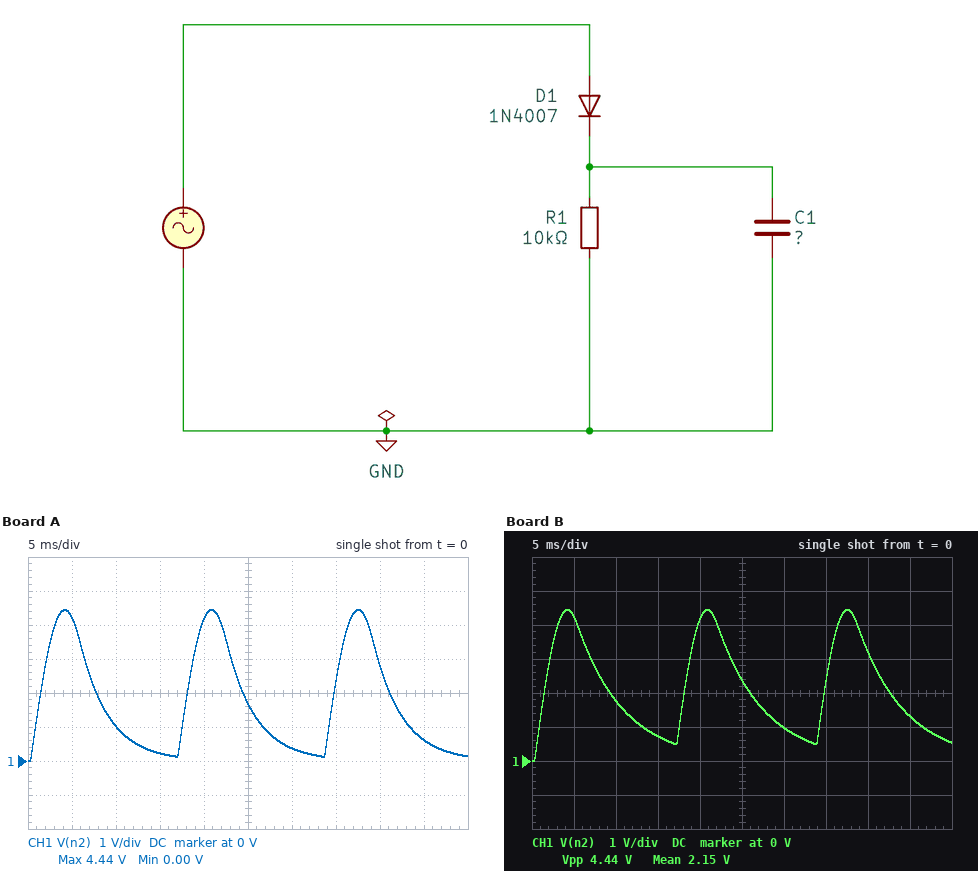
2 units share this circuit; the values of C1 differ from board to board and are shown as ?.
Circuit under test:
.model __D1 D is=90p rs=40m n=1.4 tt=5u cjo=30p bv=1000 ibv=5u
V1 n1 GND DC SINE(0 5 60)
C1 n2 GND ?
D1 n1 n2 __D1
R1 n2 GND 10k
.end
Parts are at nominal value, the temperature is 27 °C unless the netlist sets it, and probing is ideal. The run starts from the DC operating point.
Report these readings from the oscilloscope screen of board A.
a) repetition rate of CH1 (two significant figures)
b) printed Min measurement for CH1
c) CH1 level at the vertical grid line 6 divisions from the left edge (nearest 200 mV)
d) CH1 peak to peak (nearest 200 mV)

60 Hz
0.00 V
400 mV
4.4 V
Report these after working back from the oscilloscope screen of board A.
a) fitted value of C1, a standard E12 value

330 nF
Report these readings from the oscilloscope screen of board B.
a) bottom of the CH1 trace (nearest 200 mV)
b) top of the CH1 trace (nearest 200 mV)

0 V
4.4 V
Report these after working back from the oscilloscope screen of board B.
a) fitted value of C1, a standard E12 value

560 nF
